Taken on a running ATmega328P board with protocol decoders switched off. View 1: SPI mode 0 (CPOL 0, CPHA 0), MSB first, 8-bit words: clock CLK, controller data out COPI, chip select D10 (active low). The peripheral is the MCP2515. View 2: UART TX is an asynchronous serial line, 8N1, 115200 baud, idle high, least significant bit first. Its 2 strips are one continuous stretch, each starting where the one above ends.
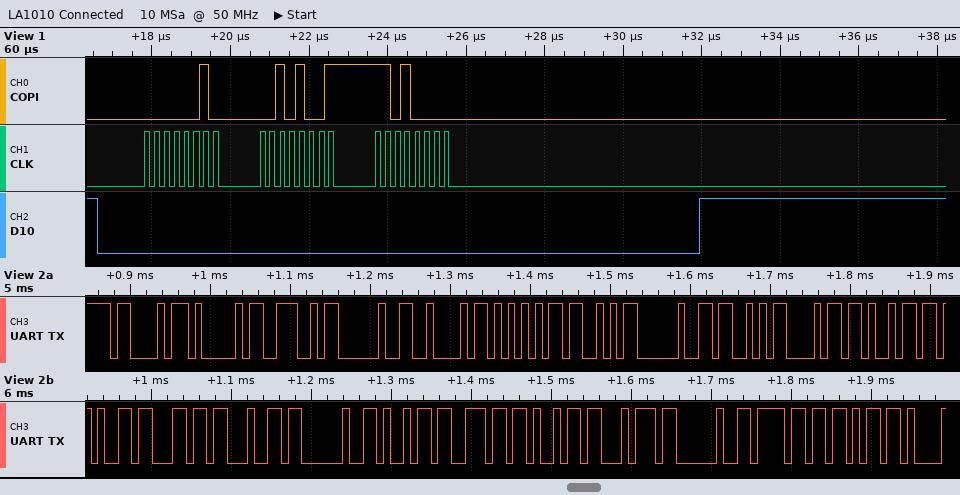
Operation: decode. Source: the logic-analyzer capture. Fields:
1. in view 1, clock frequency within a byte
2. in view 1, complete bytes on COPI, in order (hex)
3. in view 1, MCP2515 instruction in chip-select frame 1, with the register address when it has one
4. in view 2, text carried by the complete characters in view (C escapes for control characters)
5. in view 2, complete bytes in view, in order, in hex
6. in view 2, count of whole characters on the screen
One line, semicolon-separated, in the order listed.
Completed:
4 MHz; 02 29 D0; WRITE 0x29; "CAN BUS Shield init ok"; 43 41 4E 20 42 55 53 20 53 68 69 65 6C 64 20 69 6E 69 74 20 6F 6B; 22
